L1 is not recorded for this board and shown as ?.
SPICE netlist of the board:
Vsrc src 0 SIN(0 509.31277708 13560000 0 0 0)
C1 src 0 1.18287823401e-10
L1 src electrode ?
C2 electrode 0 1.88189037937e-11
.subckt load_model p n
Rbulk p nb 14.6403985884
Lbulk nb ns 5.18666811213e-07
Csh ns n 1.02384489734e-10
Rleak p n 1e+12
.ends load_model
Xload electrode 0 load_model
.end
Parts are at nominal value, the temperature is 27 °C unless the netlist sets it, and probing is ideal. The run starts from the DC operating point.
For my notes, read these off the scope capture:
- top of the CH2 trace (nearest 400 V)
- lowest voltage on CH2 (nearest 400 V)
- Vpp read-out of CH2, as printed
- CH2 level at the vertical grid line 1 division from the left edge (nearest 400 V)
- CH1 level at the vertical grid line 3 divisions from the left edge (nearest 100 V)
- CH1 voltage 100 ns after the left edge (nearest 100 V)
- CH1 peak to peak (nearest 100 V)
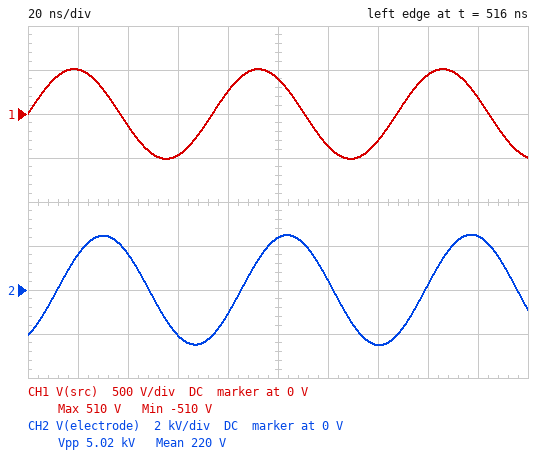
2.4 kV
-2.4 kV
5.02 kV
1.6 kV
-500 V
400 V
1.0 kV
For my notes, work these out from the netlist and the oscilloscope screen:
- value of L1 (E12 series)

680 nH
